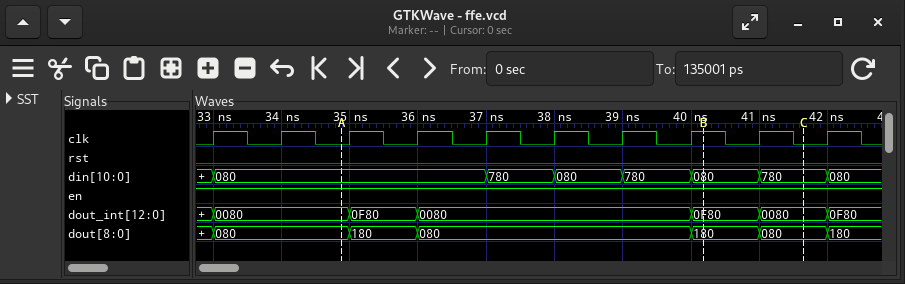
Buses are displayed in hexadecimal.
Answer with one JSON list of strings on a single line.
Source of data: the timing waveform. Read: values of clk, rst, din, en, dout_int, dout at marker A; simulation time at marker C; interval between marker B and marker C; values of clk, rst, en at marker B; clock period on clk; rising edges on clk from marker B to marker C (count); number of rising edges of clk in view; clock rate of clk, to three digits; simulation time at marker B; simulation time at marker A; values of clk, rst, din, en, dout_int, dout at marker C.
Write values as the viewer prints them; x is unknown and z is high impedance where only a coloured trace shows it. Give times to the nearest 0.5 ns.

["clk=0, rst=0, din=080, en=1, dout_int=0080, dout=080", "41.5 ns", "1.5 ns", "clk=1, rst=0, en=1", "1 ns", "1", "10", "1.00 GHz", "40 ns", "35 ns", "clk=0, rst=0, din=780, en=1, dout_int=0080, dout=080"]
